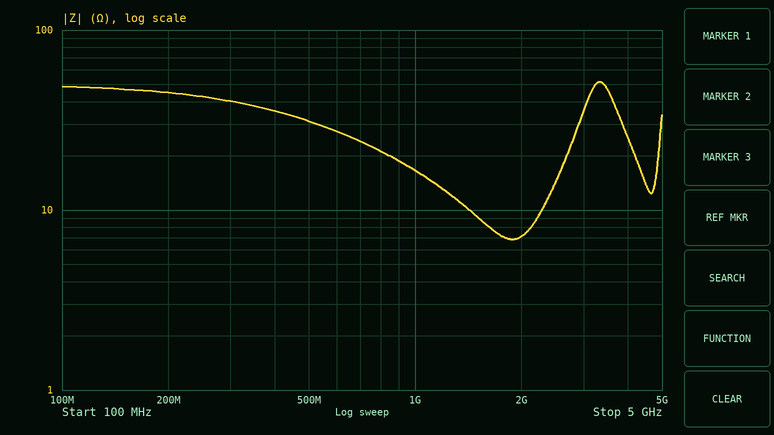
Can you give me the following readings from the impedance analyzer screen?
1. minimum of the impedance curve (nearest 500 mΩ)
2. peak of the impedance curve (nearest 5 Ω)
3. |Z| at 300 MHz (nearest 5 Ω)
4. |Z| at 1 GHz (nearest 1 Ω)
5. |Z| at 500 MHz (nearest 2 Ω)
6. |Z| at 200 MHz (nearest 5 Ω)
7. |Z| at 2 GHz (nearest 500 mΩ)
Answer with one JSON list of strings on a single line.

["7.0 Ω", "50 Ω", "40 Ω", "17 Ω", "32 Ω", "45 Ω", "7.0 Ω"]
